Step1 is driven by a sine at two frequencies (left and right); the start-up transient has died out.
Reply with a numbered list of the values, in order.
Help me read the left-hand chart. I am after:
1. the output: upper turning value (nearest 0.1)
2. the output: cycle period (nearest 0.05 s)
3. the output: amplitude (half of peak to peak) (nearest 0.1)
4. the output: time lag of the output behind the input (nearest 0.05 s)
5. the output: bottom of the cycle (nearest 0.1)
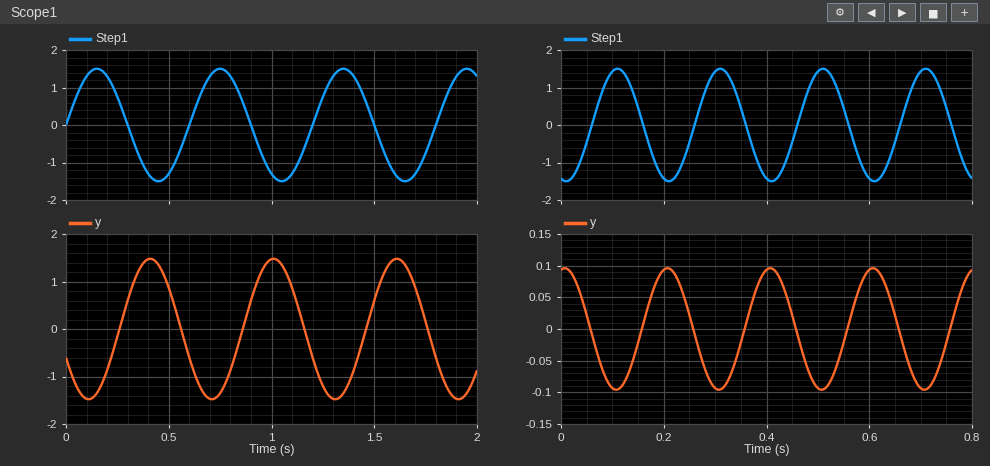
1. 1.5
2. 0.60 s
3. 1.5
4. 0.25 s
5. -1.5
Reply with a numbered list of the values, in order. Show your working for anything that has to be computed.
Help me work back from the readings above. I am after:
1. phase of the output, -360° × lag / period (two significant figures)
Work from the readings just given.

1. -360 × 0.25 / 0.6 = -150°
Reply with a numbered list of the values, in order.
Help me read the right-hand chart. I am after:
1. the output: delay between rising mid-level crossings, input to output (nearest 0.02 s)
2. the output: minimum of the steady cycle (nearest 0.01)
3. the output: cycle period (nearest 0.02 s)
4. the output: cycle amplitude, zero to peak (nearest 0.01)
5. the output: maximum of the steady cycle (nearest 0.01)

1. 0.10 s
2. -0.10
3. 0.20 s
4. 0.10
5. 0.10
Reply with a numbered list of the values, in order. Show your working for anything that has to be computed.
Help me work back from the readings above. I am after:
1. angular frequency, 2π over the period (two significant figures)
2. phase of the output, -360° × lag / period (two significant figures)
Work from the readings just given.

1. 2π / 0.2 = 31 rad/s
2. -360 × 0.1 / 0.2 = -180°
